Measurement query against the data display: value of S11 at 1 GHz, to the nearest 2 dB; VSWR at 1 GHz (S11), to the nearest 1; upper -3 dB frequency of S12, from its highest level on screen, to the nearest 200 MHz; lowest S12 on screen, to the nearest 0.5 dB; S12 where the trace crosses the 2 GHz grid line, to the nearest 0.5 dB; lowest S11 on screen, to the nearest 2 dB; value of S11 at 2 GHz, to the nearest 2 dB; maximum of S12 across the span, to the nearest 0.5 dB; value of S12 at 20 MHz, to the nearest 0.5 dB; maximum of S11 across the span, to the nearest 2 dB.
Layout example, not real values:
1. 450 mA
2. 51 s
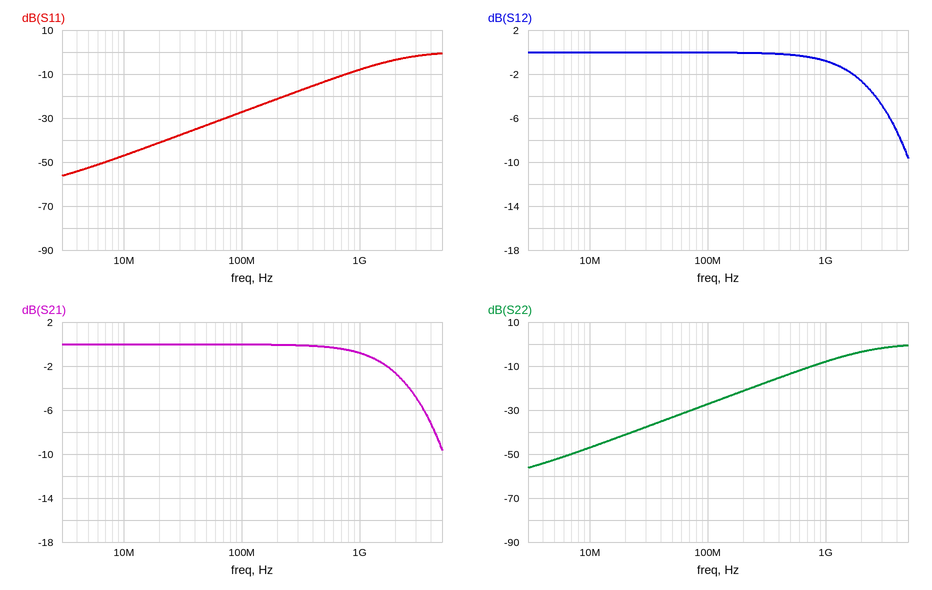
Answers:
1. -8 dB
2. 2
3. 2.2 GHz
4. -9.5 dB
5. -2.5 dB
6. -56 dB
7. -4 dB
8. 0.0 dB
9. 0.0 dB
10. 0 dB
